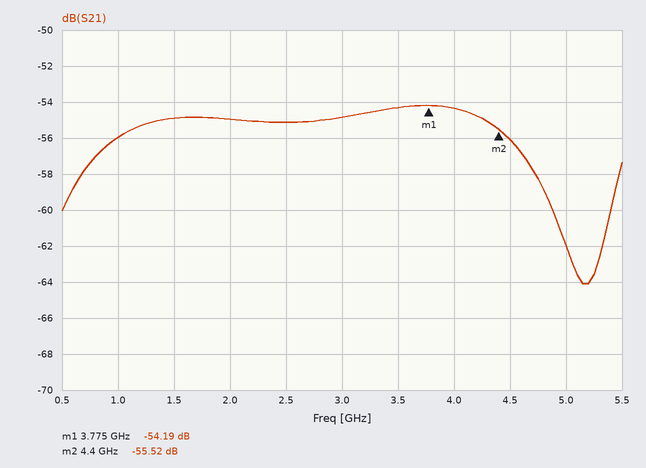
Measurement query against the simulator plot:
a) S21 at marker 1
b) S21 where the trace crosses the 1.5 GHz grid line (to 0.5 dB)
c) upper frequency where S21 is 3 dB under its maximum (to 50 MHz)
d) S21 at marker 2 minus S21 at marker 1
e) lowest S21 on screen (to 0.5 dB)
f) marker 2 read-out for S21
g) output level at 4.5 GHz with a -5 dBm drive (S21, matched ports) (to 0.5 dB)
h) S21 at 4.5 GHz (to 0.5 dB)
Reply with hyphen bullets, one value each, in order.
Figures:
- -54.19 dB
- -55.0 dB
- 4.65 GHz
- -1.33 dB
- -64.0 dB
- -55.52 dB
- -61.0 dBm
- -56.0 dB
